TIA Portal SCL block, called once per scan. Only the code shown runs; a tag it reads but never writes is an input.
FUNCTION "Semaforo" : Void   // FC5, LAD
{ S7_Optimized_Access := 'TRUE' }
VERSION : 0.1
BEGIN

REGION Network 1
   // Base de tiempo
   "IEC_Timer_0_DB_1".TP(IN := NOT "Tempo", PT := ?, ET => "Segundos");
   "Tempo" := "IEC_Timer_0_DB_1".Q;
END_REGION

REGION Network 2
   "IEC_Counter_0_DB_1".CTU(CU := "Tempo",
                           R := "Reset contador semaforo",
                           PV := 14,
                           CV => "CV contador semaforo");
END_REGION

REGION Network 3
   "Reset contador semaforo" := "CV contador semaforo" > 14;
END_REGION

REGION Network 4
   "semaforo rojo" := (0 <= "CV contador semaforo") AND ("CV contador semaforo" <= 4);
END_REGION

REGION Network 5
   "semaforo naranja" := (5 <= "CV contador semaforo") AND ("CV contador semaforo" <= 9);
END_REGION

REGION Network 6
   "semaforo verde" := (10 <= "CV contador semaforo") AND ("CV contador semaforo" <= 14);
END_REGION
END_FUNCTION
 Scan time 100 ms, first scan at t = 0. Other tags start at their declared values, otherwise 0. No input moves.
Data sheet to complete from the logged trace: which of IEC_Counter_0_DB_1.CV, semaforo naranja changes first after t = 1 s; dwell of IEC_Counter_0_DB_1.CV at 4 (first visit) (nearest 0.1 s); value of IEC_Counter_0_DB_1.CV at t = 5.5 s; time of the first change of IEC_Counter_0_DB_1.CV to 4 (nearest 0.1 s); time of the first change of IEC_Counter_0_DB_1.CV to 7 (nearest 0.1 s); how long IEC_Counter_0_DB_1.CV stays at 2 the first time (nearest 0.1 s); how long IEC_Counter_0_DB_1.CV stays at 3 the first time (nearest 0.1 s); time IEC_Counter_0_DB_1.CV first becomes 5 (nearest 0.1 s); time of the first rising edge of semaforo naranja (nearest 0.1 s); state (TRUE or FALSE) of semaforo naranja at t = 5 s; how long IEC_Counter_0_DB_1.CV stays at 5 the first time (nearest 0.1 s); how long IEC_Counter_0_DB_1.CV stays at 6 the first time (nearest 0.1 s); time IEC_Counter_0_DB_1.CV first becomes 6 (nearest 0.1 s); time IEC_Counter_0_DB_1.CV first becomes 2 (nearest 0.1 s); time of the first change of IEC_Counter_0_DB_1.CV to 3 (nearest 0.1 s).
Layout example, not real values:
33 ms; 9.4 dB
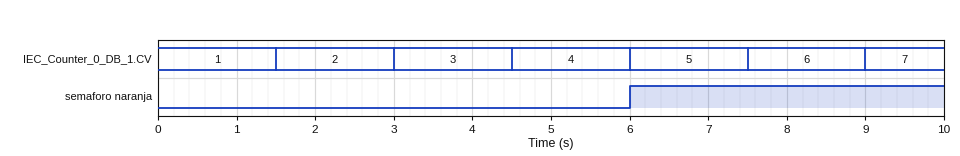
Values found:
IEC_Counter_0_DB_1.CV; 1.5 s; 4; 4.5 s; 9.0 s; 1.5 s; 1.5 s; 6.0 s; 6.0 s; FALSE; 1.5 s; 1.5 s; 7.5 s; 1.5 s; 3.0 s
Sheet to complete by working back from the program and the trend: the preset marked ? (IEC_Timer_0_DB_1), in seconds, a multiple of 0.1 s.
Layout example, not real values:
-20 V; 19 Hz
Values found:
1.4 s
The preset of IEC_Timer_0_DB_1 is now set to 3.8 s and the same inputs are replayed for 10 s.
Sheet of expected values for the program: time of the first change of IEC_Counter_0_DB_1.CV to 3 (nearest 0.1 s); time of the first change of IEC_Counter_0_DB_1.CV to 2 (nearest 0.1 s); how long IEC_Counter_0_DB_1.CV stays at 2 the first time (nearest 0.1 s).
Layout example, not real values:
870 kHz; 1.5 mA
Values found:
7.8 s; 3.9 s; 3.9 s
